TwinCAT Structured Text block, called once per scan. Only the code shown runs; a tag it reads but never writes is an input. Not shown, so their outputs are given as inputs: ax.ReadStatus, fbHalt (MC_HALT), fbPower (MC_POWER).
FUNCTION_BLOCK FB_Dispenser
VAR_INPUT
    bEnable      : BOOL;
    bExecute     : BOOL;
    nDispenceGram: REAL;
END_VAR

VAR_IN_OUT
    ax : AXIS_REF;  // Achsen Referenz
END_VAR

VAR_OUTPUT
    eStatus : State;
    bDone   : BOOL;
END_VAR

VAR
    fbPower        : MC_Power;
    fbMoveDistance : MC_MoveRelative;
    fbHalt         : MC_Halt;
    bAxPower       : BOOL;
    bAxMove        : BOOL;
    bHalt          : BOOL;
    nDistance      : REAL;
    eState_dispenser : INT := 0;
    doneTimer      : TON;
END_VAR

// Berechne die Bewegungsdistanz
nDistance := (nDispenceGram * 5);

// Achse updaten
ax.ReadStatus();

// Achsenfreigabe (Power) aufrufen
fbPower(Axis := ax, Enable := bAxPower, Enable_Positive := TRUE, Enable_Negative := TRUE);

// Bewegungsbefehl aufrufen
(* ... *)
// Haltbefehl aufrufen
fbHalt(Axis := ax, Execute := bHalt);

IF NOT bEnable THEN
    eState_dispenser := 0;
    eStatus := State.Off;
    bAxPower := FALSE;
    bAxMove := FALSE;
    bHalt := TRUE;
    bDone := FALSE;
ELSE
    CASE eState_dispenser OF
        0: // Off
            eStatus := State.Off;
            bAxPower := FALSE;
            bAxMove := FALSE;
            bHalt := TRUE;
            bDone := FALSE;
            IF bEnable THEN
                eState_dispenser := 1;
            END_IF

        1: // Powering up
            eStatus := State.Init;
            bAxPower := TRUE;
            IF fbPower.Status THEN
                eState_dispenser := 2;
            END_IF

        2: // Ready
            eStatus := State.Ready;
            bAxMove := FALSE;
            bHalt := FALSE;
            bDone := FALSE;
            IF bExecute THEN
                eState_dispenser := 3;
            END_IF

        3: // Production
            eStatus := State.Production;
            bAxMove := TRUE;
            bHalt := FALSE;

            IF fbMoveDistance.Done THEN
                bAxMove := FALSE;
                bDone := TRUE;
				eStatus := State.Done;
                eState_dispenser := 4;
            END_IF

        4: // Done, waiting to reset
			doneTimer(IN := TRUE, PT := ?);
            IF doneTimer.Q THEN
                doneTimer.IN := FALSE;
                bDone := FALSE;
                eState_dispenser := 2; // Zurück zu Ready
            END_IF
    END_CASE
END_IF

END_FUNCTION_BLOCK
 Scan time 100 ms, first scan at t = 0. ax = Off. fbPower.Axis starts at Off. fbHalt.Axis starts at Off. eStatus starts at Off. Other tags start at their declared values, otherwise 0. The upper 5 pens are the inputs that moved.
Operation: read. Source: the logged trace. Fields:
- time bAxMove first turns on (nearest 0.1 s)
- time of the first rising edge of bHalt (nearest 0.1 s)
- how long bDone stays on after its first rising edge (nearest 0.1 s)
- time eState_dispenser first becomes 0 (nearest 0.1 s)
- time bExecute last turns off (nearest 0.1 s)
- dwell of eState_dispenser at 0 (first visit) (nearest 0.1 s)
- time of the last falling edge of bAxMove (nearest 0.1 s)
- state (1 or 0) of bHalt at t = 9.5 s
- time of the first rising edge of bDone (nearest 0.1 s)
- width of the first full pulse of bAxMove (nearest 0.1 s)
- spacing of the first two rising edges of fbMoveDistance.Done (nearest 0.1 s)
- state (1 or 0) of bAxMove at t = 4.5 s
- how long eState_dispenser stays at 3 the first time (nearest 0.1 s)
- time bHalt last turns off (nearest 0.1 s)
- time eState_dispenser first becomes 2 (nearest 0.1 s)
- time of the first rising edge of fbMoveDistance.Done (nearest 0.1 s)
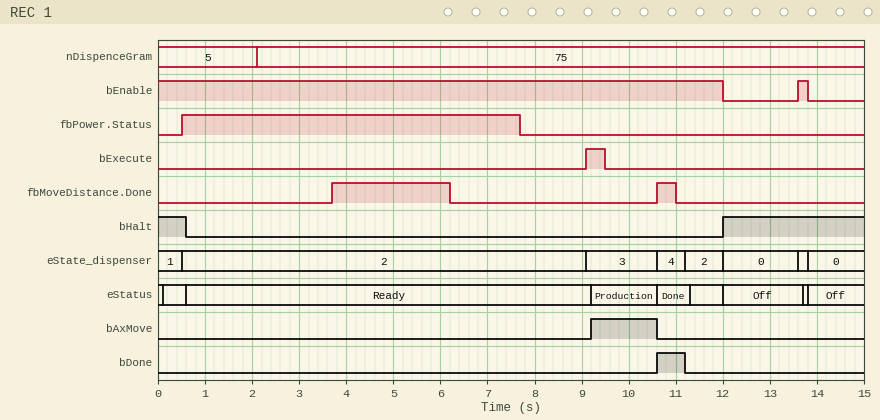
9.2 s
12.0 s
0.6 s
12.0 s
9.5 s
1.6 s
10.6 s
0
10.6 s
1.4 s
6.9 s
0
1.5 s
0.6 s
0.5 s
3.7 s
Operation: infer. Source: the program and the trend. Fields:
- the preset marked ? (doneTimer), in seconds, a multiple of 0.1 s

0.5 s
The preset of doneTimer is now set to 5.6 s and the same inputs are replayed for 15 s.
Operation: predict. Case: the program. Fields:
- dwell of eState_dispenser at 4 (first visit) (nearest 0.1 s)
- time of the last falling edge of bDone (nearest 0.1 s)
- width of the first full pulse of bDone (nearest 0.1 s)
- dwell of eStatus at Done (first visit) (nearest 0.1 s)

1.4 s
12.0 s
1.4 s
1.4 s
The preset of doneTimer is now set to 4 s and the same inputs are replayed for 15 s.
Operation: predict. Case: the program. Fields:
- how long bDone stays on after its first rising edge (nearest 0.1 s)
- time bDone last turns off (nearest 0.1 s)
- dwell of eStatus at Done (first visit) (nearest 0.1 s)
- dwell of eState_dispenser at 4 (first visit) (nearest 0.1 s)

1.4 s
12.0 s
1.4 s
1.4 s
